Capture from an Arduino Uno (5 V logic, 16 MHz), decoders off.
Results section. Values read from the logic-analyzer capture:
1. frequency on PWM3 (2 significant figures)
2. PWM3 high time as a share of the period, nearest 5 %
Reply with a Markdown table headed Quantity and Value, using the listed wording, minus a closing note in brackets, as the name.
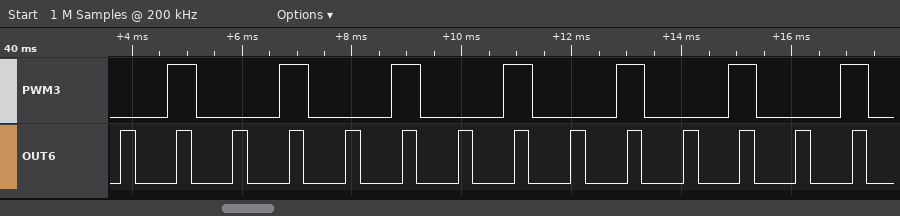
| Quantity | Value |
|---|---|
| frequency on PWM3 | 490 Hz |
| PWM3 high time as a share of the period, nearest 5 % | 25 % |
